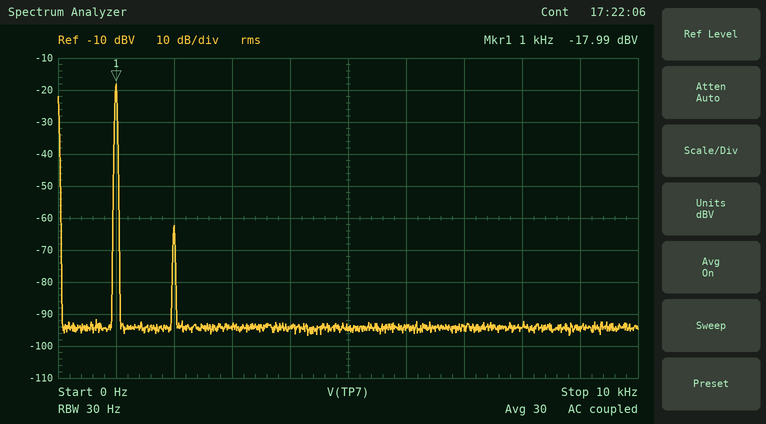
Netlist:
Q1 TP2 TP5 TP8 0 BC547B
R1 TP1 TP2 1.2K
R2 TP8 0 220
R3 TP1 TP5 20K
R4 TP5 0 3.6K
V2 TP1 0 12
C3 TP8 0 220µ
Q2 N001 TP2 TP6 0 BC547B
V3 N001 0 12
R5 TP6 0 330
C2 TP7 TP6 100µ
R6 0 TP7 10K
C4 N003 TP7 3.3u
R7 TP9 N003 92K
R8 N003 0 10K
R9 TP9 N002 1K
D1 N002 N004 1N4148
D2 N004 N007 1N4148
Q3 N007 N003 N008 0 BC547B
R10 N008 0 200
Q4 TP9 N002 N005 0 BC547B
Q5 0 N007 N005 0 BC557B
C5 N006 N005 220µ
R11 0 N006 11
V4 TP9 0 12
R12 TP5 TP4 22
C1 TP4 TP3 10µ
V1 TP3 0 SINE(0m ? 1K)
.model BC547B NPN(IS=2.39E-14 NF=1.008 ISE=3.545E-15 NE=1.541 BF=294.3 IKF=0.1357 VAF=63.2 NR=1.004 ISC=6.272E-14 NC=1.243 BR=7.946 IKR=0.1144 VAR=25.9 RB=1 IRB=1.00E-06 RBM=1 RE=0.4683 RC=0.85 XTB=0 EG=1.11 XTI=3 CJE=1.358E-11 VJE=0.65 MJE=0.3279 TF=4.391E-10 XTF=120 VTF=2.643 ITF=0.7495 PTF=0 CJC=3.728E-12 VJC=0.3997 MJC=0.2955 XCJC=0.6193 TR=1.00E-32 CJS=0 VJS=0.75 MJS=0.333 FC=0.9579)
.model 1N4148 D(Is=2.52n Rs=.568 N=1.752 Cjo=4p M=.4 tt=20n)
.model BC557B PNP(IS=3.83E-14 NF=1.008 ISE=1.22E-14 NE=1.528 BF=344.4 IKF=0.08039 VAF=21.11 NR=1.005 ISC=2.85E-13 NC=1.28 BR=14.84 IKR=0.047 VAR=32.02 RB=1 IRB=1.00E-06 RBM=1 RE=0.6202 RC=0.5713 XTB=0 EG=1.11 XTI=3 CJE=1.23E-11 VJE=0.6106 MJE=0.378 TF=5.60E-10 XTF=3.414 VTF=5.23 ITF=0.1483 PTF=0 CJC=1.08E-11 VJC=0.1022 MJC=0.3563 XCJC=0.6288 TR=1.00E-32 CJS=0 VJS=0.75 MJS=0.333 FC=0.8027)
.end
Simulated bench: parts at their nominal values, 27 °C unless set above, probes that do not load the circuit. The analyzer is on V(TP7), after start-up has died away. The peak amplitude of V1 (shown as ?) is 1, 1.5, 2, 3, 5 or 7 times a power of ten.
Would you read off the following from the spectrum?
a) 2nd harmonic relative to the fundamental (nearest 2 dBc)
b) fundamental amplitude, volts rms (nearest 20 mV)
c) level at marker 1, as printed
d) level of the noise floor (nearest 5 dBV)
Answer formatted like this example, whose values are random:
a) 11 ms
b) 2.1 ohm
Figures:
a) -44 dBc
b) 120 mV
c) -17.99 dBV
d) -95 dBV
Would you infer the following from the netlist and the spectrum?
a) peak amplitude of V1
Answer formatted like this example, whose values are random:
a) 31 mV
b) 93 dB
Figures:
a) 1 mV
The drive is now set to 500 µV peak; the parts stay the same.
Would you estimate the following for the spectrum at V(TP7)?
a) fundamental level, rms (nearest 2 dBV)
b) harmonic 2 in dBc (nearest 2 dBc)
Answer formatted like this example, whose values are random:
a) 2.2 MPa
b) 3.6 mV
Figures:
a) -24 dBV
b) -50 dBc
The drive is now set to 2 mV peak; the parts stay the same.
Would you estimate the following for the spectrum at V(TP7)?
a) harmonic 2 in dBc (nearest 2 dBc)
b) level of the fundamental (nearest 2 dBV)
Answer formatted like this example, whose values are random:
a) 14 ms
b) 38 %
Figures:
a) -38 dBc
b) -12 dBV
